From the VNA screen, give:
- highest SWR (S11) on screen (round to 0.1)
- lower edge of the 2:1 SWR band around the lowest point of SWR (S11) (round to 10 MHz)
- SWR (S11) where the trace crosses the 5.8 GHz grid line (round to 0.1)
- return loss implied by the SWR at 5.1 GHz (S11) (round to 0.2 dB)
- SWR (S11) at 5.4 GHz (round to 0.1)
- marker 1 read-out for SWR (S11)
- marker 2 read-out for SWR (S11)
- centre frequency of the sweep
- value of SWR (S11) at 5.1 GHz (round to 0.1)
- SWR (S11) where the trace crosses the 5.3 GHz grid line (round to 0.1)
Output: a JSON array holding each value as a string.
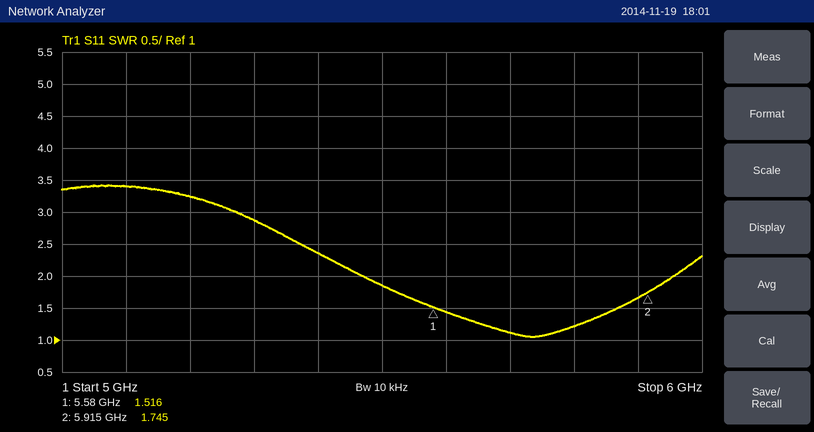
["3.4", "5.47 GHz", "1.2", "5.2 dB", "2.4", "1.516", "1.745", "5.5 GHz", "3.4", "2.9"]
